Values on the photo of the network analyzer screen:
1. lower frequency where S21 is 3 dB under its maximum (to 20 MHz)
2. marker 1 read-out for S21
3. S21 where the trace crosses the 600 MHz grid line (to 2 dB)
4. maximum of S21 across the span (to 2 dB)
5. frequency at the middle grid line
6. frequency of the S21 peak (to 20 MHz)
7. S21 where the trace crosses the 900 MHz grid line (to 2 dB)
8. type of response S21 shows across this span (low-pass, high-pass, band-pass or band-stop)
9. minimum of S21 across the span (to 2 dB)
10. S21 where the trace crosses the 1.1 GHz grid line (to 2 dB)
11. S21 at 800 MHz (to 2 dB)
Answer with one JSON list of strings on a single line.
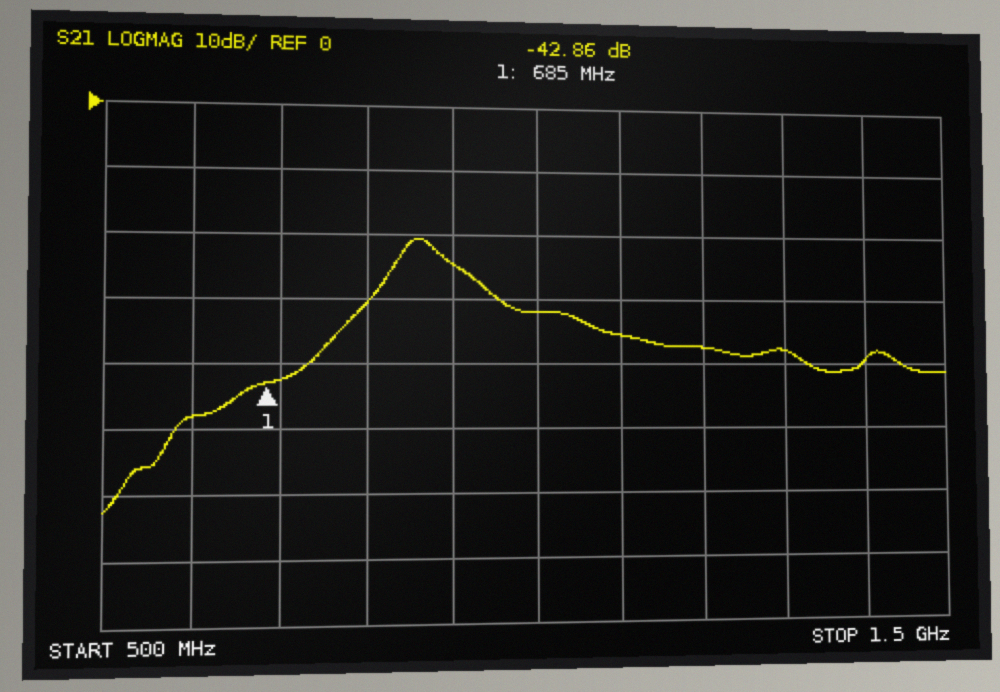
["840 MHz", "-42.86 dB", "-48 dB", "-20 dB", "1 GHz", "860 MHz", "-24 dB", "band-pass", "-62 dB", "-36 dB", "-30 dB"]
